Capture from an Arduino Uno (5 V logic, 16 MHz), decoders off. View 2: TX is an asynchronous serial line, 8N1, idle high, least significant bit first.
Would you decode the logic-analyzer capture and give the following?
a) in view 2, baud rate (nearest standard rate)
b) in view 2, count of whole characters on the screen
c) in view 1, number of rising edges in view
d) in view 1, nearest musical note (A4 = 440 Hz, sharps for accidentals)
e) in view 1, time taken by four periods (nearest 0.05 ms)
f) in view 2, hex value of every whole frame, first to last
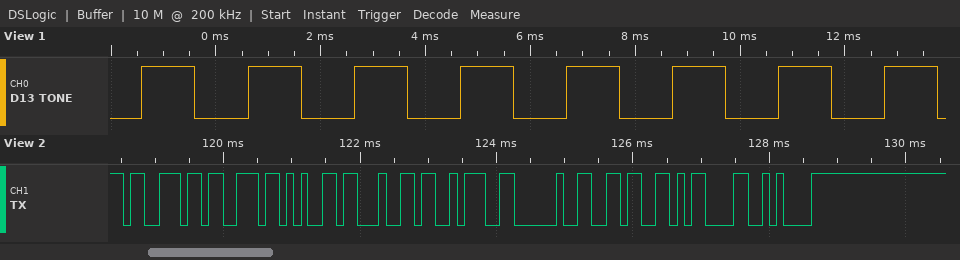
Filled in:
9600 baud
9
8
B4
8.10 ms
73 73 65 64 3A 20 36 0D 0A
